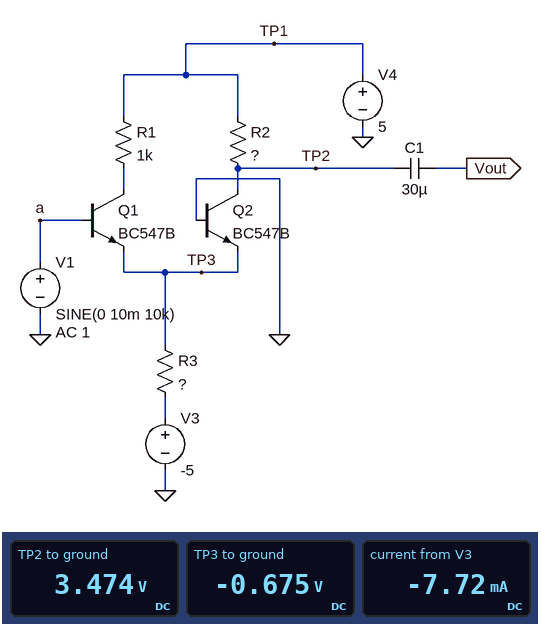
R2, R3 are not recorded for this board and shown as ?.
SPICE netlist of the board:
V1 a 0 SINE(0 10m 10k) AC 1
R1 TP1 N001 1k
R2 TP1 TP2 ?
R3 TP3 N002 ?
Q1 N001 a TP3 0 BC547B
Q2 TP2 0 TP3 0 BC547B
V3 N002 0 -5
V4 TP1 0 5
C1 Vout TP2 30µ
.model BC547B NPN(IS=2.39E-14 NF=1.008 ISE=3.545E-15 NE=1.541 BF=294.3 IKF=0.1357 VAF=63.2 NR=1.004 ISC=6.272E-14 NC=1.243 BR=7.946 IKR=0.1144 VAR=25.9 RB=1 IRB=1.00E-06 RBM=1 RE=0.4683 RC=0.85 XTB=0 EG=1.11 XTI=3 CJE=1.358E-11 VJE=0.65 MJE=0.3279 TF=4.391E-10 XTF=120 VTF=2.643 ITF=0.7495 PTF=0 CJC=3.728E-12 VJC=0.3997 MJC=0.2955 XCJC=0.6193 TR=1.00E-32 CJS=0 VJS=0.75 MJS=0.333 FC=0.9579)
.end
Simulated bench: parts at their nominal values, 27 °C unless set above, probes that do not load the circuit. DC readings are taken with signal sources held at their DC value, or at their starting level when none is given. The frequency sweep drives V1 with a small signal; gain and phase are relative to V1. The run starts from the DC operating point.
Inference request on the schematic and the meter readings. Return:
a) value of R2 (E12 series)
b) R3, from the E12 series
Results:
390 Ω
560 Ω
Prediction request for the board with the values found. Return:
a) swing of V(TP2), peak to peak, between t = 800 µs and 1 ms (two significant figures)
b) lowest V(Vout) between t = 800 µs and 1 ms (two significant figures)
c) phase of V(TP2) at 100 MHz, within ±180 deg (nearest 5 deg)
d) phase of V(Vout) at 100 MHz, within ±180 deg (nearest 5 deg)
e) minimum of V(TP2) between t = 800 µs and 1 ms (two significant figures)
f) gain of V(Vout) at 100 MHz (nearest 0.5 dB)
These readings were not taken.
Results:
500 mV
-250 mV
-30 deg
-30 deg
3.2 V
27.0 dB
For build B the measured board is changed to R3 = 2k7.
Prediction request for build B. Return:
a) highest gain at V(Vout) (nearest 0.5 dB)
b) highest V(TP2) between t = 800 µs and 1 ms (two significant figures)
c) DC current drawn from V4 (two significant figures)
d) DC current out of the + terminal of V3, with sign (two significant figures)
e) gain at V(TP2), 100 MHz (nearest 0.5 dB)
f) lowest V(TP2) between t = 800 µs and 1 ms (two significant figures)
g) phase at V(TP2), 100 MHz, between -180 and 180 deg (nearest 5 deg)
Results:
15.5 dB
4.7 V
1.6 mA
-1.6 mA
14.5 dB
4.6 V
-25 deg
